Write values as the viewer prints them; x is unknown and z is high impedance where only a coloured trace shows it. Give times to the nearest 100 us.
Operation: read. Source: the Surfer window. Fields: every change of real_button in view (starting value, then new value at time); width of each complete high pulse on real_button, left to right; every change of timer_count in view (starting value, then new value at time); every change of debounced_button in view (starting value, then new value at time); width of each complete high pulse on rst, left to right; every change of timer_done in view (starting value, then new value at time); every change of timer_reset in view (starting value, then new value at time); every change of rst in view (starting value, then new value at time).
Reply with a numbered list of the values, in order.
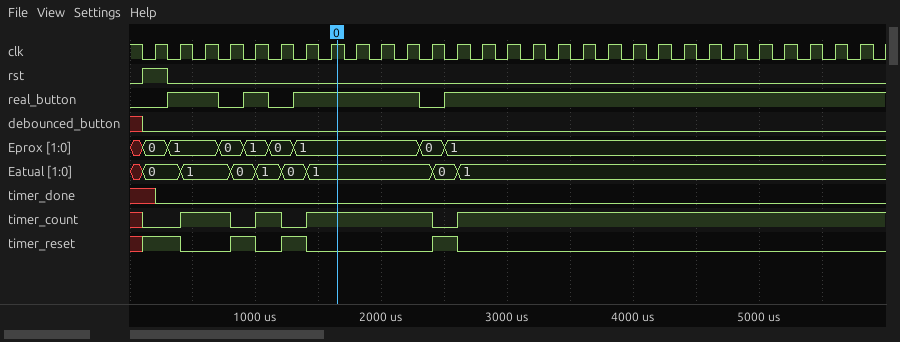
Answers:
1. 0, 1 at 300 us, 0 at 700 us, 1 at 900 us, 0 at 1100 us, 1 at 1300 us, 0 at 2300 us, 1 at 2500 us
2. 400 us, 200 us, 1000 us
3. x, 0 at 100 us, 1 at 400 us, 0 at 800 us, 1 at 1000 us, 0 at 1200 us, 1 at 1400 us, 0 at 2400 us, 1 at 2600 us
4. x, 0 at 100 us
5. 200 us
6. x, 0 at 200 us
7. x, 1 at 100 us, 0 at 400 us, 1 at 800 us, 0 at 1000 us, 1 at 1200 us, 0 at 1400 us, 1 at 2400 us, 0 at 2600 us
8. 0, 1 at 100 us, 0 at 300 us
